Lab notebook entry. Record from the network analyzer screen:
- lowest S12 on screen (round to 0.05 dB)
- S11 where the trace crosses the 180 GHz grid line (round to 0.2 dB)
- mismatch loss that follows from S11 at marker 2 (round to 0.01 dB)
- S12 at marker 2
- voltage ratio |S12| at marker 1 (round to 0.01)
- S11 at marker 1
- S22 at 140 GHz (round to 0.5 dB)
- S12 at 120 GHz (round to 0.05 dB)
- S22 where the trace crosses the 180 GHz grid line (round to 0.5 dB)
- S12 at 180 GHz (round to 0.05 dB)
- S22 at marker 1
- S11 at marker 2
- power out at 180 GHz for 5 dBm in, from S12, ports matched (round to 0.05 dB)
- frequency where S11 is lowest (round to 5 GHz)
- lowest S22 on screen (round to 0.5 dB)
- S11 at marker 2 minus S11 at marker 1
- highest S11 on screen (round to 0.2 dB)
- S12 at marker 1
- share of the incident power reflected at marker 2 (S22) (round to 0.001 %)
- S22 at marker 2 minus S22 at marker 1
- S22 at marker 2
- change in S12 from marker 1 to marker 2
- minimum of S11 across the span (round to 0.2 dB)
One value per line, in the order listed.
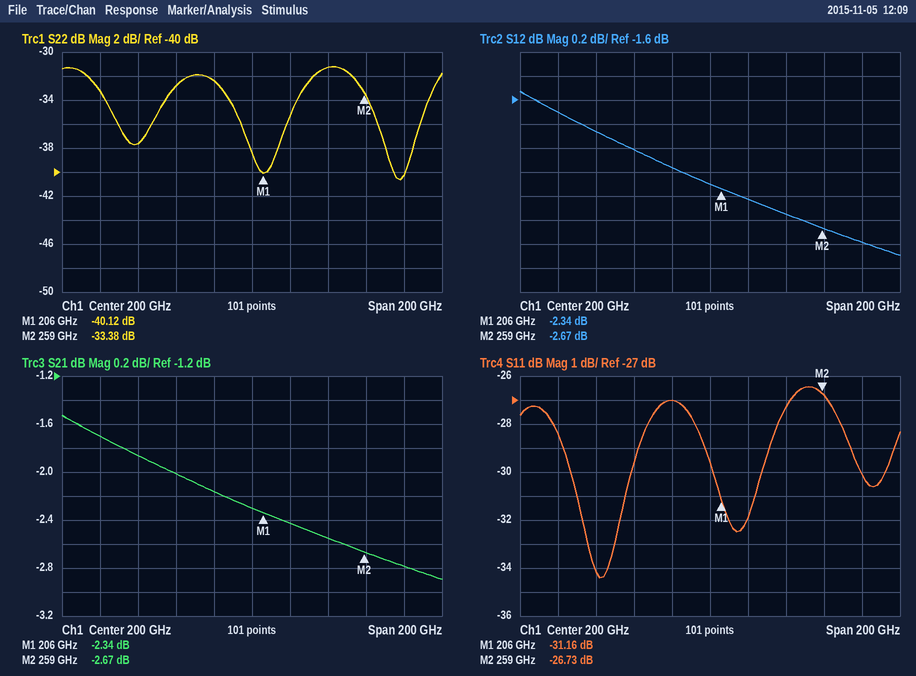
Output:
-2.90 dB
-27.0 dB
0.01 dB
-2.67 dB
0.76
-31.16 dB
-37.5 dB
-1.70 dB
-32.5 dB
-2.15 dB
-40.12 dB
-26.73 dB
2.85 dBm
140 GHz
-40.5 dB
4.43 dB
-26.4 dB
-2.34 dB
0.046 %
6.74 dB
-33.38 dB
-0.33 dB
-34.4 dB
